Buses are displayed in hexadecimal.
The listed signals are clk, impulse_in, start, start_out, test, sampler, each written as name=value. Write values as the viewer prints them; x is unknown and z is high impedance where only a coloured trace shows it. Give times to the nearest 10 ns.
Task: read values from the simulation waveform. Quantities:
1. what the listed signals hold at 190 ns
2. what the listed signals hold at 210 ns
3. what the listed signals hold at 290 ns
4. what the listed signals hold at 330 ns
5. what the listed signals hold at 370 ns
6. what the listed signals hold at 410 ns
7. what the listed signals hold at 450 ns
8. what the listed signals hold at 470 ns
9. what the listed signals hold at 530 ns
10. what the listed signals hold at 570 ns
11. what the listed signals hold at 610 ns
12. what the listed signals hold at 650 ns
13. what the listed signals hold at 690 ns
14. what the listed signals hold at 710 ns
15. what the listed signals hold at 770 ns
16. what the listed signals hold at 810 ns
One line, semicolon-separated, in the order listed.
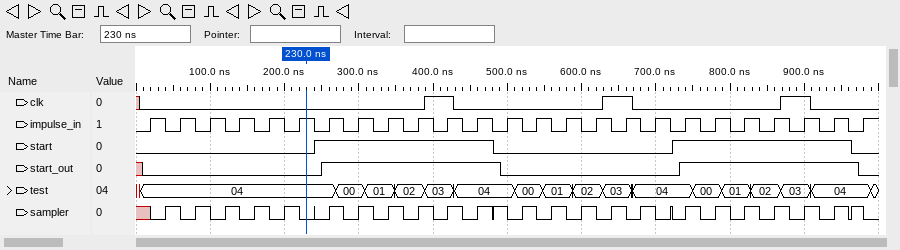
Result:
clk=0, impulse_in=1, start=0, start_out=0, test=04, sampler=0; clk=0, impulse_in=0, start=0, start_out=0, test=04, sampler=1; clk=0, impulse_in=0, start=1, start_out=1, test=00, sampler=0; clk=0, impulse_in=0, start=1, start_out=1, test=01, sampler=0; clk=0, impulse_in=0, start=1, start_out=1, test=02, sampler=0; clk=1, impulse_in=0, start=1, start_out=1, test=03, sampler=0; clk=0, impulse_in=0, start=1, start_out=1, test=04, sampler=0; clk=0, impulse_in=1, start=1, start_out=1, test=04, sampler=1; clk=0, impulse_in=0, start=0, start_out=0, test=00, sampler=1; clk=0, impulse_in=0, start=0, start_out=0, test=01, sampler=1; clk=0, impulse_in=0, start=0, start_out=0, test=02, sampler=1; clk=1, impulse_in=0, start=0, start_out=0, test=03, sampler=1; clk=0, impulse_in=0, start=0, start_out=0, test=04, sampler=1; clk=0, impulse_in=1, start=0, start_out=0, test=04, sampler=0; clk=0, impulse_in=0, start=1, start_out=1, test=00, sampler=0; clk=0, impulse_in=0, start=1, start_out=1, test=01, sampler=0
